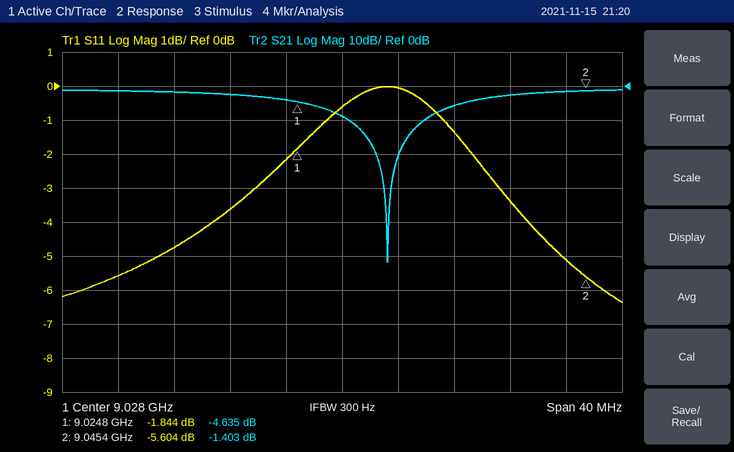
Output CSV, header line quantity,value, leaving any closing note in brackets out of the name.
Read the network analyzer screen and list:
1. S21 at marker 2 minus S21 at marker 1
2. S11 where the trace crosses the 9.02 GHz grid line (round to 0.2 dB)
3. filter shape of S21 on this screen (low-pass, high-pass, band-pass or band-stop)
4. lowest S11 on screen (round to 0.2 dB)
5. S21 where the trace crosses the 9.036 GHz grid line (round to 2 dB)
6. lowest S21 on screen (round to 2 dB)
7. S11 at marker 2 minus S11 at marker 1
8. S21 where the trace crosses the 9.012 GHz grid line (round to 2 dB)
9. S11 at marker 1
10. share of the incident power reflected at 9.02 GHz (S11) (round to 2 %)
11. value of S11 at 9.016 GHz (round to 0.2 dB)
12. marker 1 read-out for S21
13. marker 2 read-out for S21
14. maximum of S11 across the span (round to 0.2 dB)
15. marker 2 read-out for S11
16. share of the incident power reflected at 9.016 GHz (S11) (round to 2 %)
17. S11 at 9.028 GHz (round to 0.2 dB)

quantity,value
S21 at marker 2 minus S21 at marker 1,3.232 dB
S11 where the trace crosses the 9.02 GHz grid line,-3.6 dB
filter shape of S21 on this screen,band-stop
lowest S11 on screen,-6.4 dB
S21 where the trace crosses the 9.036 GHz grid line,-6 dB
lowest S21 on screen,-52 dB
S11 at marker 2 minus S11 at marker 1,-3.760 dB
S21 where the trace crosses the 9.012 GHz grid line,-2 dB
S11 at marker 1,-1.844 dB
share of the incident power reflected at 9.02 GHz (S11),44 %
value of S11 at 9.016 GHz,-4.8 dB
marker 1 read-out for S21,-4.635 dB
marker 2 read-out for S21,-1.403 dB
maximum of S11 across the span,0.0 dB
marker 2 read-out for S11,-5.604 dB
share of the incident power reflected at 9.016 GHz (S11),34 %
S11 at 9.028 GHz,-0.6 dB
